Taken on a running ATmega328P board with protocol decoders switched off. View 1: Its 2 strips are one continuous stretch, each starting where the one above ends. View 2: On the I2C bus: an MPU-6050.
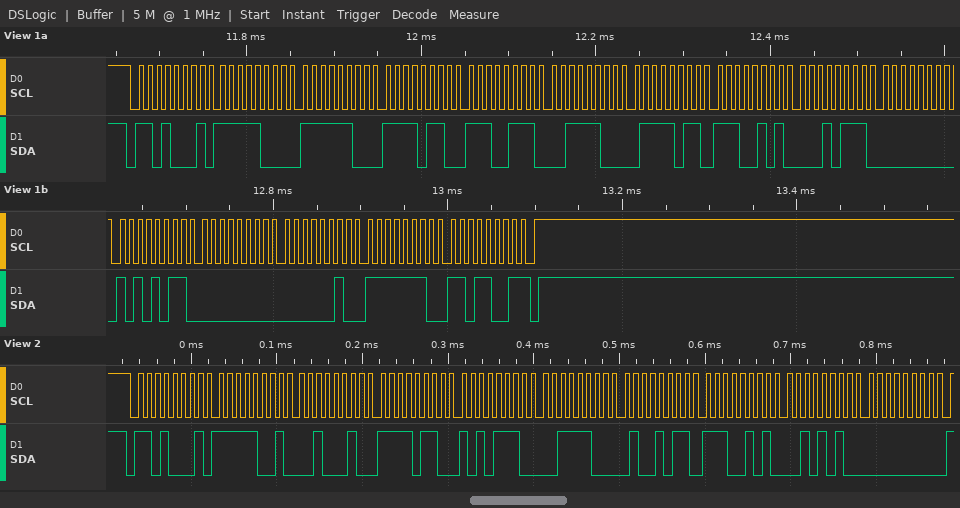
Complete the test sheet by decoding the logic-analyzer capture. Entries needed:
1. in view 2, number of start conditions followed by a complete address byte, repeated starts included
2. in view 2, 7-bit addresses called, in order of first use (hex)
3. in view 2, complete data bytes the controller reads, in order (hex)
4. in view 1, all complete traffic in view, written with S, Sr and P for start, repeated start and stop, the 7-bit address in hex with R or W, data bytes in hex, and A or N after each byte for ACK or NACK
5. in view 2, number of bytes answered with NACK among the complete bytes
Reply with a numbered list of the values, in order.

1. 1
2. 0x68
3. F9 22 F6 AE 3C 4B E5 2A 00
4. S 68R A F8 A FC A F6 A E7 A 3C A 7B A E5 A 17 A 00 A AB A 00 A 02 A FE A D9 N P
5. 0
